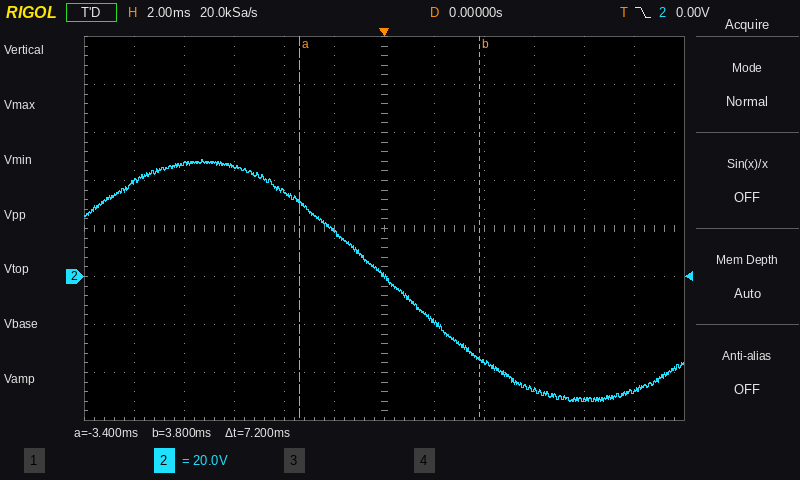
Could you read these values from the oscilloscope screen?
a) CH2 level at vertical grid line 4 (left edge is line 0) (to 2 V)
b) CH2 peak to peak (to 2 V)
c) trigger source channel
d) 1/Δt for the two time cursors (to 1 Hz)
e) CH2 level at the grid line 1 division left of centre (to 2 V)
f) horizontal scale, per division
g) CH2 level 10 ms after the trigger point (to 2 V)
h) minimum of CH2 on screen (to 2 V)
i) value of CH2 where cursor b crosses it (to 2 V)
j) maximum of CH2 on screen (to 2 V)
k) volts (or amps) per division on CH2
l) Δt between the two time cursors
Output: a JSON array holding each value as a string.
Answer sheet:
["36 V", "100 V", "CH2", "139 Hz", "18 V", "2 ms", "-48 V", "-52 V", "-34 V", "48 V", "20 V", "7.2 ms"]
